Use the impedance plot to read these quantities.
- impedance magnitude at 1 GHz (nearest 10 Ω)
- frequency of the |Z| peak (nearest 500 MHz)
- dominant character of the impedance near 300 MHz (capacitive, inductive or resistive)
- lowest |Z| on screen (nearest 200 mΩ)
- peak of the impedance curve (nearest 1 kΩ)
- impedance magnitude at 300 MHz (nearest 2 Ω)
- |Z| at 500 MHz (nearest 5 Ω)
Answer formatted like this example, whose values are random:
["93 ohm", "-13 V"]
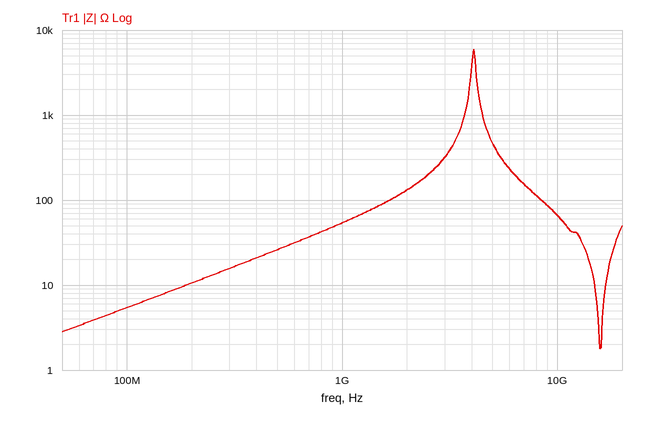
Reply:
["50 Ω", "4.0 GHz", "inductive", "1.8 Ω", "6 kΩ", "16 Ω", "25 Ω"]
